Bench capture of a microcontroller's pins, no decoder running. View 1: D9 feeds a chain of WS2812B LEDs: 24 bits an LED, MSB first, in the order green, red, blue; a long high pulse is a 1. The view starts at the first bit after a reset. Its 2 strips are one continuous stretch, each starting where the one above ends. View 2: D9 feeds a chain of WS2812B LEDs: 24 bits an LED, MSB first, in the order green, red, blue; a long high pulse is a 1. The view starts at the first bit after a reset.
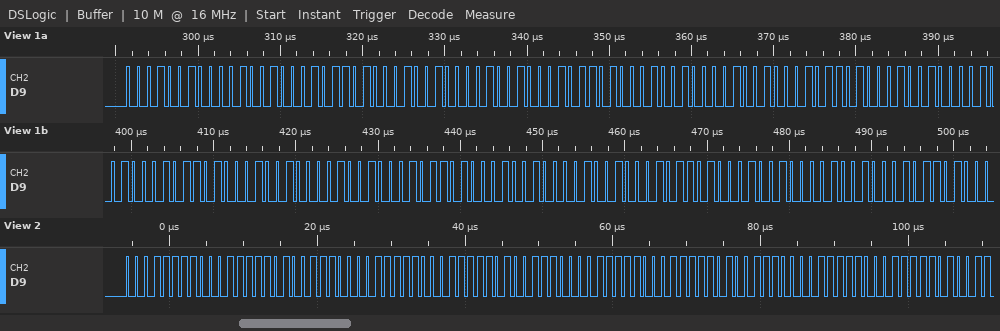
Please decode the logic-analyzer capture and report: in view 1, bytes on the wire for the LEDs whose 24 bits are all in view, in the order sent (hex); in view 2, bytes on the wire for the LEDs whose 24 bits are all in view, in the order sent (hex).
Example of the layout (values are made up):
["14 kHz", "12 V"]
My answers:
["12 12 2D 12 12 2D 12 12 2D 12 12 2D 12 12 2D 12 12 2D 12 12 2D", "1F 1F 4E 1F 1F 4E 1F 1F 4E"]
